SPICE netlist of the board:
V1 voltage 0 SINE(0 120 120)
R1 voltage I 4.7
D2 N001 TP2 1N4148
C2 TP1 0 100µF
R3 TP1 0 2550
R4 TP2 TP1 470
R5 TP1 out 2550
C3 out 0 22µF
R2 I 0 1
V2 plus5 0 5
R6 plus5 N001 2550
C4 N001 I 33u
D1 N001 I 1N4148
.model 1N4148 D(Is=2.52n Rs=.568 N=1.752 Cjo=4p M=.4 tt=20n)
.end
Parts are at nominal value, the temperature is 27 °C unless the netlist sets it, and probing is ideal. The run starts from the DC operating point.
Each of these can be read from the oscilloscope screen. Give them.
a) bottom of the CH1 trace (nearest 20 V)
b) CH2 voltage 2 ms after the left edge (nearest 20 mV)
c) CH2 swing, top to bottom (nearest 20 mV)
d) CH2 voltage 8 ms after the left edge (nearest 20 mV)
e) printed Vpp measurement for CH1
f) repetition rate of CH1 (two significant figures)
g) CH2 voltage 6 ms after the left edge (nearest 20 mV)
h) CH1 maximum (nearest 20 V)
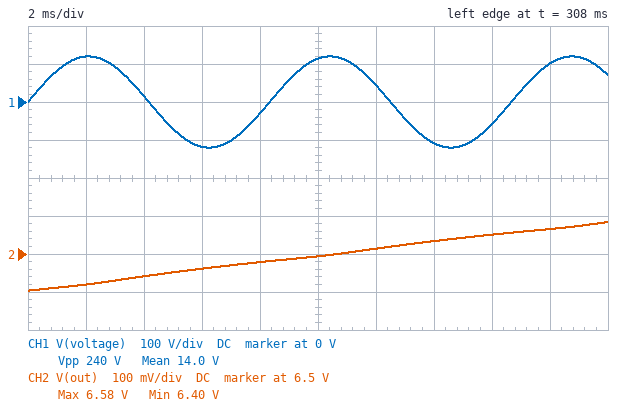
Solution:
-120 V
6.42 V
180 mV
6.48 V
240 V
120 Hz
6.46 V
120 V
